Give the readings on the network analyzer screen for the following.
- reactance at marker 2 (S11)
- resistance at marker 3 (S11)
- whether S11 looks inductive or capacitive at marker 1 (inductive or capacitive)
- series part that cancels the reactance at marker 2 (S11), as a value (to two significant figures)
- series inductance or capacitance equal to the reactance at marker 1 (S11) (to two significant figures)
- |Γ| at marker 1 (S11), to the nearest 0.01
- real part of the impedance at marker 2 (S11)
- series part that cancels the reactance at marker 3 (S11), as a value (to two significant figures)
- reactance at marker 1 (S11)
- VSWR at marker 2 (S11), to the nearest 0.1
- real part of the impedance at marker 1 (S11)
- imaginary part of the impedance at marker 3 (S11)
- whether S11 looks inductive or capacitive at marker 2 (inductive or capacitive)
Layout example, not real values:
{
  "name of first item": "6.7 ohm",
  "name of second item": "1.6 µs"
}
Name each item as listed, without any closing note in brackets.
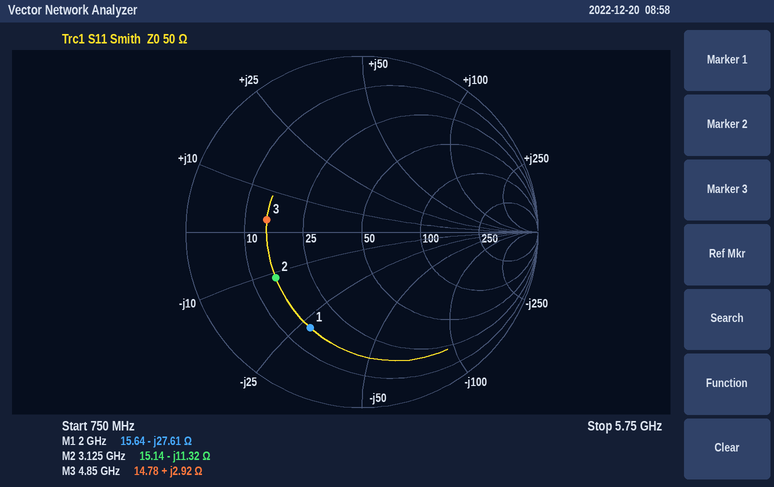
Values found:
{
  "reactance at marker 2": "-11.32 Ω",
  "resistance at marker 3": "14.78 Ω",
  "whether S11 looks inductive or capacitive at marker 1": "capacitive",
  "series part that cancels the reactance at marker 2 (S11), as a value": "580 pH",
  "series inductance or capacitance equal to the reactance at marker 1 (S11)": "2.9 pF",
  "|Γ| at marker 1 (S11), to the nearest 0.01": "0.62",
  "real part of the impedance at marker 2": "15.14 Ω",
  "series part that cancels the reactance at marker 3 (S11), as a value": "11 pF",
  "reactance at marker 1": "-27.61 Ω",
  "VSWR at marker 2 (S11), to the nearest 0.1": "3.5",
  "real part of the impedance at marker 1": "15.64 Ω",
  "imaginary part of the impedance at marker 3": "+2.92 Ω",
  "whether S11 looks inductive or capacitive at marker 2": "capacitive"
}
